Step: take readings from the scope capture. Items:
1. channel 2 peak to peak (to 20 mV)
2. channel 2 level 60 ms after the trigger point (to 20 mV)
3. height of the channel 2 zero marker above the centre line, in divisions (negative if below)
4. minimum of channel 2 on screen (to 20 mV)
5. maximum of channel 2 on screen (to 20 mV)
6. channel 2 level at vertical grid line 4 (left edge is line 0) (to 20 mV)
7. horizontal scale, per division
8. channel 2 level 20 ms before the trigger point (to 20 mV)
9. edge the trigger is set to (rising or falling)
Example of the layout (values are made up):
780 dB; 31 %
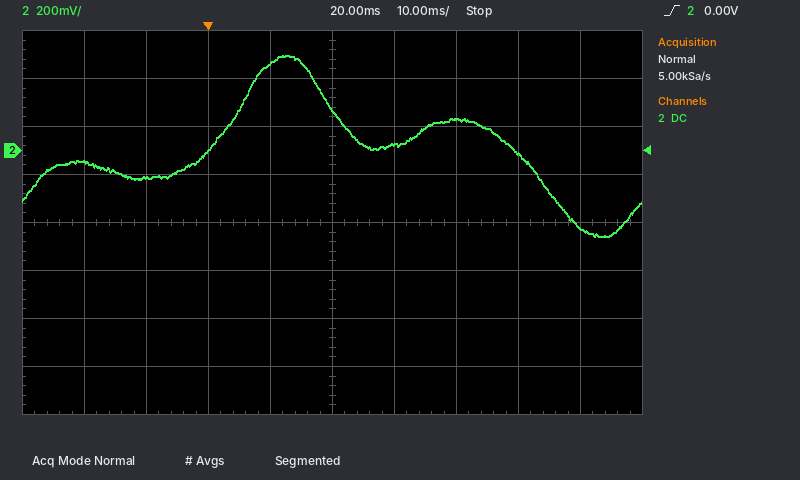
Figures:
760 mV; -320 mV; +1.5 div; -360 mV; 400 mV; 360 mV; 10 ms; -40 mV; rising
